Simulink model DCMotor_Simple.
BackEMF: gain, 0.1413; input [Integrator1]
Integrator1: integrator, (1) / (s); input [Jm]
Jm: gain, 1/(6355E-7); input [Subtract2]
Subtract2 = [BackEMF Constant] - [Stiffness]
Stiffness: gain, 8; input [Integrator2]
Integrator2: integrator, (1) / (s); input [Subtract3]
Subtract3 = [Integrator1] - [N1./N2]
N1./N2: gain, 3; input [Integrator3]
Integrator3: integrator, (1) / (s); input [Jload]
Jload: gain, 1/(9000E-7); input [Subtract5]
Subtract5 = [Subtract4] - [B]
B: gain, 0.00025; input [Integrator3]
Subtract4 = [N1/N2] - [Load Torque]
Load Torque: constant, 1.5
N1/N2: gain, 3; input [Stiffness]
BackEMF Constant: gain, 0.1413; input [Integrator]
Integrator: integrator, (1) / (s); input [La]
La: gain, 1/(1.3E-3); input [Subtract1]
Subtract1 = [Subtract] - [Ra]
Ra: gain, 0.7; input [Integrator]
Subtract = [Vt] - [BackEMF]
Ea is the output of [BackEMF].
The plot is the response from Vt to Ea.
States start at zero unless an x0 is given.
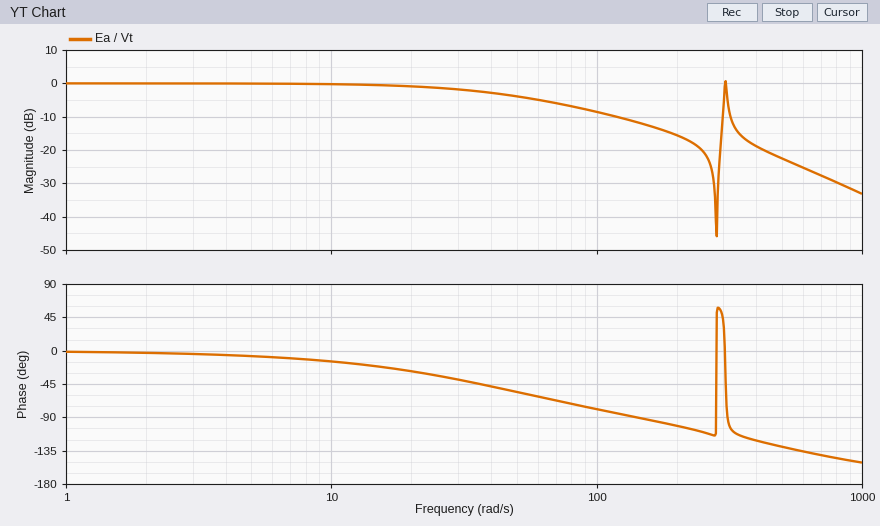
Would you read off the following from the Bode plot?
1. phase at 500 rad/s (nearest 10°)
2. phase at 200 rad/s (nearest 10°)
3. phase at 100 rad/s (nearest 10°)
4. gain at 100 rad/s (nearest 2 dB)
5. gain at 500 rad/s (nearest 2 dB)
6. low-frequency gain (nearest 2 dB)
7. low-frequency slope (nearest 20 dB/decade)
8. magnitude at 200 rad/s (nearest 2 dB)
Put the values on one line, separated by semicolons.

-130°; -100°; -80°; -8 dB; -22 dB; 0 dB; 0 dB/decade; -16 dB
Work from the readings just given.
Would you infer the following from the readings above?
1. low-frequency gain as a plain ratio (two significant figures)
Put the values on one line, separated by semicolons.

1.0
